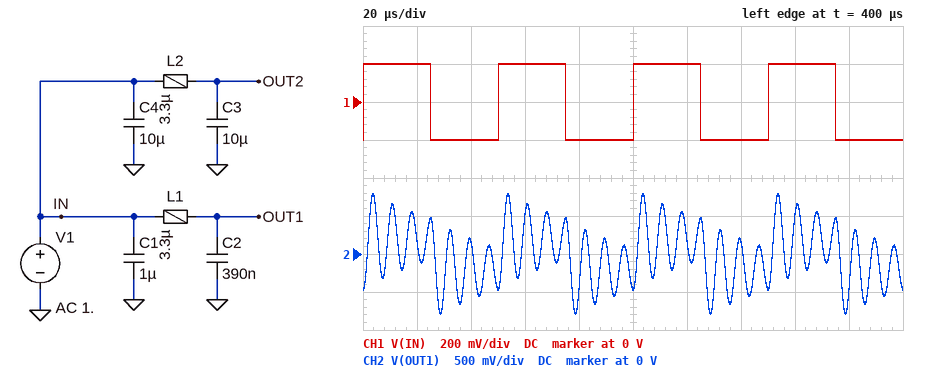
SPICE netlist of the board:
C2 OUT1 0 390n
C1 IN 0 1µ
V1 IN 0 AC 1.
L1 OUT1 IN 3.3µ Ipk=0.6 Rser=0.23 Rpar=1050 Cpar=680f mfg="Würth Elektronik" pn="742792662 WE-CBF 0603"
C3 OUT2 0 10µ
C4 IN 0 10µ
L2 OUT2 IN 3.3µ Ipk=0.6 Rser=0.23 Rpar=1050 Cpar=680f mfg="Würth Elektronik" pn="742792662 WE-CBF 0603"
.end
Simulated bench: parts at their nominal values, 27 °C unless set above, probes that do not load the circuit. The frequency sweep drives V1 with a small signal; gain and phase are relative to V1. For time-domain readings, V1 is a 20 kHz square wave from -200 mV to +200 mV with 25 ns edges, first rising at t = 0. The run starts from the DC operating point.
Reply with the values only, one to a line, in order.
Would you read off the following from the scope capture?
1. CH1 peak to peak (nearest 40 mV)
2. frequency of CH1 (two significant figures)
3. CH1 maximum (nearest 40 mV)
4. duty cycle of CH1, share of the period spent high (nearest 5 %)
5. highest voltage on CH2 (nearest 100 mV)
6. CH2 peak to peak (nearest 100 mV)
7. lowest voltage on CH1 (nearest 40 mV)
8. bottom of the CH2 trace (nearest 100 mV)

400 mV
20 kHz
200 mV
50 %
800 mV
1.6 V
-200 mV
-800 mV
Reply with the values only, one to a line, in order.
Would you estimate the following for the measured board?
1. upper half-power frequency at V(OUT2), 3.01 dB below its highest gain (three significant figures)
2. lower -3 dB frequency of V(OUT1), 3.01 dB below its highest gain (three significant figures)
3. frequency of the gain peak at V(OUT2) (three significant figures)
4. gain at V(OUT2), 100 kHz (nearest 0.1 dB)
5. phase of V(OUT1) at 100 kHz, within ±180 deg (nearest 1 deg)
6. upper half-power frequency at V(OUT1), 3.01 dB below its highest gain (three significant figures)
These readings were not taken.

31.7 kHz
134 kHz
26.6 kHz
-21.7 dB
-7 deg
146 kHz
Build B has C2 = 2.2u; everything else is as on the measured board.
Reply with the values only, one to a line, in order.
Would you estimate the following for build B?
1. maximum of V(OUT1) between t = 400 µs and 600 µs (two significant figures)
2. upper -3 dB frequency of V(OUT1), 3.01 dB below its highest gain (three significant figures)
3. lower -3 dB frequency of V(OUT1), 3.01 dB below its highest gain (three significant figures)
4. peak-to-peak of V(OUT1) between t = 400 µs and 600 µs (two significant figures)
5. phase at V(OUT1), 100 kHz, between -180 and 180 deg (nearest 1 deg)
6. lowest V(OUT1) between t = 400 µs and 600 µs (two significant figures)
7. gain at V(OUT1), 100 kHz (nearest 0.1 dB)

690 mV
63.9 kHz
52.6 kHz
1.4 V
-170 deg
-690 mV
-5.5 dB
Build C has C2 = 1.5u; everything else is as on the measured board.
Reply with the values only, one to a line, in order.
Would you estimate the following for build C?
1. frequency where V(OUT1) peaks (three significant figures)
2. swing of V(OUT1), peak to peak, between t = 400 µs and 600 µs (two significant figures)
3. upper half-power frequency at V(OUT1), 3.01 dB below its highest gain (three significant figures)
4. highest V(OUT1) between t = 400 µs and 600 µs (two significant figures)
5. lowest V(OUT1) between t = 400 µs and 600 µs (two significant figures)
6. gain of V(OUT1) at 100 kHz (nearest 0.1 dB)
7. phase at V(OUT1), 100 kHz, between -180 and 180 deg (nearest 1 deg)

71.1 kHz
960 mV
76.5 kHz
480 mV
-480 mV
0.2 dB
-167 deg
